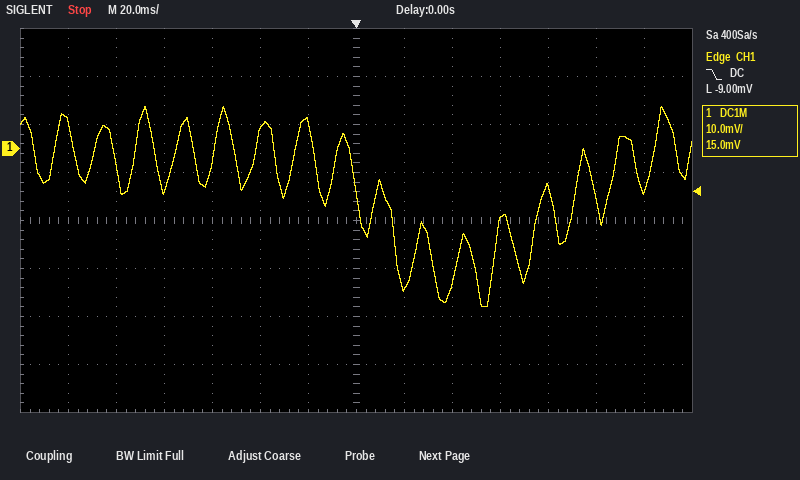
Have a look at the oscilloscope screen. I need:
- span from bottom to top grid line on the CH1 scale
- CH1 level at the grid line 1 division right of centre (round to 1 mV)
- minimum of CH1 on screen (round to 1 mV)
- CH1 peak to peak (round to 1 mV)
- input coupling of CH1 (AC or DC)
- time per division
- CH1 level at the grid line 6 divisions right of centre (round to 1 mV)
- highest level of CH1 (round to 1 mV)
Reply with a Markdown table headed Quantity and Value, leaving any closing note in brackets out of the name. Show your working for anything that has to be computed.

| Quantity | Value |
|---|---|
| span from bottom to top grid line on the CH1 scale | 80 mV |
| CH1 level at the grid line 1 division right of centre | -29 mV |
| minimum of CH1 on screen | -33 mV |
| CH1 peak to peak | 9 mV − (-33 mV) = 42 mV |
| input coupling of CH1 | DC |
| time per division | 20 ms |
| CH1 level at the grid line 6 divisions right of centre | -9 mV |
| highest level of CH1 | 9 mV |
